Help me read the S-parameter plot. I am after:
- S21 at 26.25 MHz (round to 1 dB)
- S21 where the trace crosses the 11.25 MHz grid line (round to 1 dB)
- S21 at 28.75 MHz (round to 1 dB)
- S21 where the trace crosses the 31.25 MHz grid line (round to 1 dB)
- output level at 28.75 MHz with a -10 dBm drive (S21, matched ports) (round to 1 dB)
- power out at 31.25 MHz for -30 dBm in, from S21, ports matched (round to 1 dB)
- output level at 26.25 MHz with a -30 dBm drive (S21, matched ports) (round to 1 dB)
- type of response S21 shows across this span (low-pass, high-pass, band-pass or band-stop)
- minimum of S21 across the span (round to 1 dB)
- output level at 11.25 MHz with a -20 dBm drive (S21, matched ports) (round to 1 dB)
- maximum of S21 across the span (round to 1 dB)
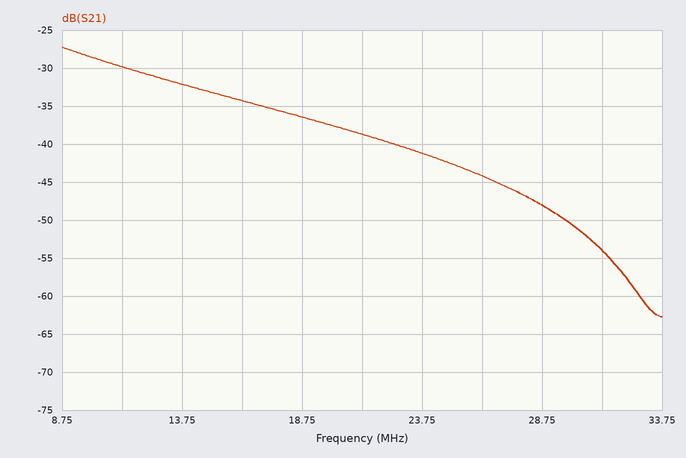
-44 dB
-30 dB
-48 dB
-54 dB
-58 dBm
-84 dBm
-74 dBm
low-pass
-63 dB
-50 dBm
-27 dB
